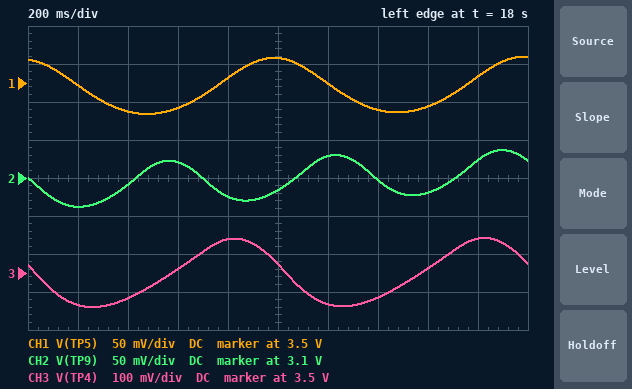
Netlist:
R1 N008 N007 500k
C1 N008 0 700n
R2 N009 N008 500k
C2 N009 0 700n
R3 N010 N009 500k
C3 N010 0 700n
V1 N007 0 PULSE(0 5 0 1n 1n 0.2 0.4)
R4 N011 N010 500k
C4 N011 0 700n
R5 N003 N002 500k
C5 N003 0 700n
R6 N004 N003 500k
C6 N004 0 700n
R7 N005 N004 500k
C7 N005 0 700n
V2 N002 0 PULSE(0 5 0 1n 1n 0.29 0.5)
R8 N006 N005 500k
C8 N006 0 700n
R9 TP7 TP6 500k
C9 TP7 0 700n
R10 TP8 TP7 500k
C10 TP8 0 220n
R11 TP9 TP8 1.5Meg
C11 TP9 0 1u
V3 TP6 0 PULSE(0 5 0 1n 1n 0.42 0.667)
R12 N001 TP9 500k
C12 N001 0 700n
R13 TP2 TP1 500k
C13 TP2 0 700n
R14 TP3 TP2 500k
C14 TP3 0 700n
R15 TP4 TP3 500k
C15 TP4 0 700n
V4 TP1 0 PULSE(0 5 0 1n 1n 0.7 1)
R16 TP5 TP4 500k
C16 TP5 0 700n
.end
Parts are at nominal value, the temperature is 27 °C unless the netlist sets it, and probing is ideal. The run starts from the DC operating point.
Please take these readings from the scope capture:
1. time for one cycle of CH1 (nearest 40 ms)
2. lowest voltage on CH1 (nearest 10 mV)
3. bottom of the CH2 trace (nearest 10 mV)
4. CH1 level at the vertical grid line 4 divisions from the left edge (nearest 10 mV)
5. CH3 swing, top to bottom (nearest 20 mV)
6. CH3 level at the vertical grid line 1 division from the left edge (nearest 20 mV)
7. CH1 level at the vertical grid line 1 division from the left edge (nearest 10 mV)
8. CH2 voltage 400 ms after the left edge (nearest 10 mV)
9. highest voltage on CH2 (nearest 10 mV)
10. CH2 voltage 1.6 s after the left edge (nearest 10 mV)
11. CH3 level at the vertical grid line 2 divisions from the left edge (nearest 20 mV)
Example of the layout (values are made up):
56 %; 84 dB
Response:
1.00 s; 3.46 V; 3.06 V; 3.51 V; 180 mV; 3.42 V; 3.50 V; 3.09 V; 3.14 V; 3.08 V; 3.44 V
